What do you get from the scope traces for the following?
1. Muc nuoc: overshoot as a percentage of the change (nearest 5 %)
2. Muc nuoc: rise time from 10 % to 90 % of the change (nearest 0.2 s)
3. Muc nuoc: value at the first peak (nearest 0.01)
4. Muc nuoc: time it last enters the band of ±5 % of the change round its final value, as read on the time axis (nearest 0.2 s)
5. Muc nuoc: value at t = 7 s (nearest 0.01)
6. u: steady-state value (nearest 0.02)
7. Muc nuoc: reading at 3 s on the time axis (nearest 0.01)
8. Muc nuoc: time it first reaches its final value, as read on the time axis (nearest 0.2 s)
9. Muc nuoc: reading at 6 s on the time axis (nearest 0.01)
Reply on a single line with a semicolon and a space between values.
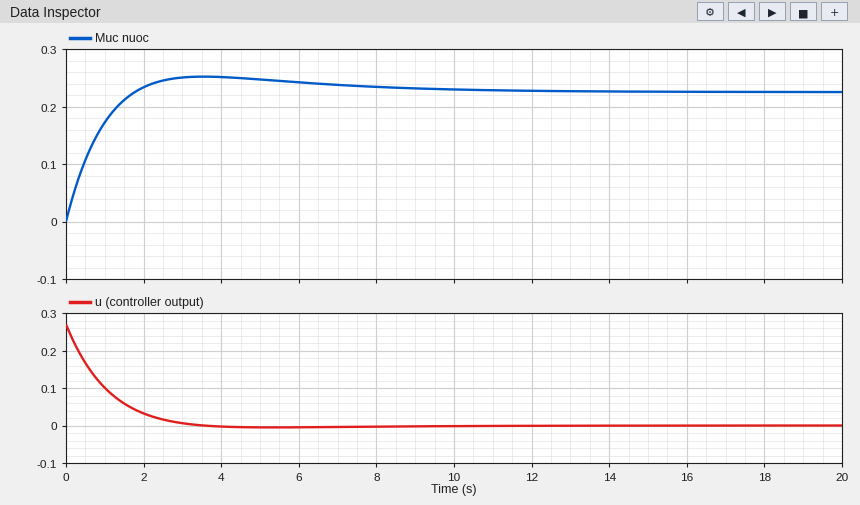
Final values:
10 %; 1.2 s; 0.25; 7.4 s; 0.24; 0.00; 0.25; 1.8 s; 0.24
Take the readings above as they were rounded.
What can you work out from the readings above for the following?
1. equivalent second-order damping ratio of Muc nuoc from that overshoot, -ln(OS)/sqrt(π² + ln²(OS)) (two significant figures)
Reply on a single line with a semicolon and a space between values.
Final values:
0.59
